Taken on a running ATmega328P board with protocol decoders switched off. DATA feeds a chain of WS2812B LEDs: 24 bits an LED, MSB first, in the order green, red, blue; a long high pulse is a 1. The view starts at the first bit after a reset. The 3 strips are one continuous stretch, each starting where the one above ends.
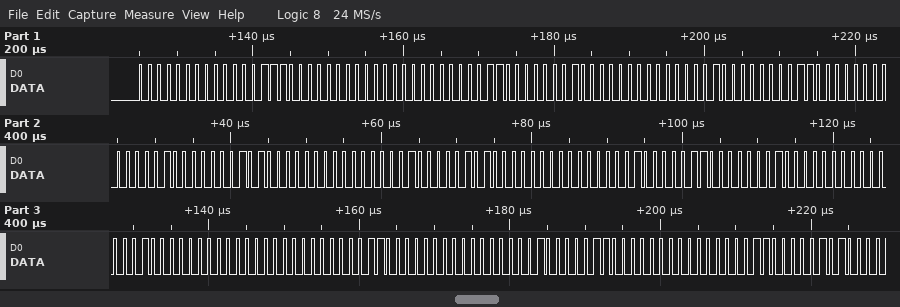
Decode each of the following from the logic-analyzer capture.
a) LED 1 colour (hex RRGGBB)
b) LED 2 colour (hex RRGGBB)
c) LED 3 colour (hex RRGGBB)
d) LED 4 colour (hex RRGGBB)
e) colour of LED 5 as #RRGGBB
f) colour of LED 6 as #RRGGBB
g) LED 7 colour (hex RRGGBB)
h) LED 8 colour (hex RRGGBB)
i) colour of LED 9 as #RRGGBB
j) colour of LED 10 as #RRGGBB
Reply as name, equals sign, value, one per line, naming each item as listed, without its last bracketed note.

LED 1 colour = #070000
LED 2 colour = #060002
LED 3 colour = #040003
LED 4 colour = #040005
colour of LED 5 as #RRGGBB = #010005
colour of LED 6 as #RRGGBB = #010006
LED 7 colour = #000204
LED 8 colour = #000006
colour of LED 9 as #RRGGBB = #010006
colour of LED 10 as #RRGGBB = #030005
